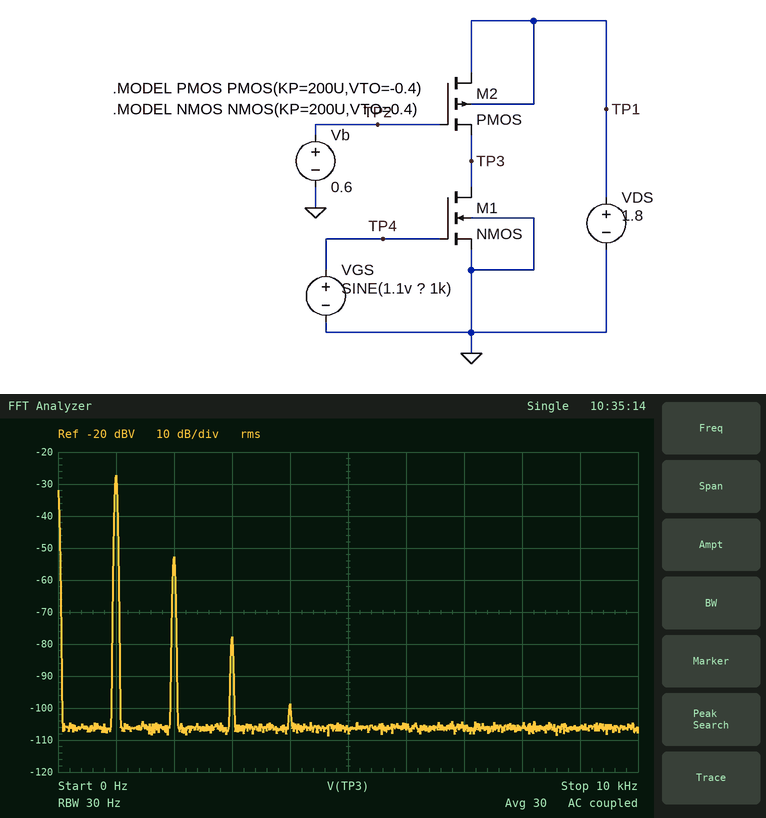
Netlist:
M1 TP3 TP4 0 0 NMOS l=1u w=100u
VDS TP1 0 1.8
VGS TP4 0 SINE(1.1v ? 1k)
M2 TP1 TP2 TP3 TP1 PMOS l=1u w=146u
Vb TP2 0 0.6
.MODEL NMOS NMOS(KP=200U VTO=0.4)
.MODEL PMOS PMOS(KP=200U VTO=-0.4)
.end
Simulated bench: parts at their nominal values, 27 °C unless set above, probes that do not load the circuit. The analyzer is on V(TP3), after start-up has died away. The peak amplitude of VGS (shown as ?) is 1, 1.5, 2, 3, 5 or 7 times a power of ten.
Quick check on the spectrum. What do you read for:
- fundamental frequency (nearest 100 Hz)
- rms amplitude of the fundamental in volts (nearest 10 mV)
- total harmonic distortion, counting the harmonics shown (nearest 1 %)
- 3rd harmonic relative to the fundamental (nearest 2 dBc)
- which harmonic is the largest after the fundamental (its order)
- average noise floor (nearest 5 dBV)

1.0 kHz
40 mV
5 %
-50 dBc
2
-105 dBV
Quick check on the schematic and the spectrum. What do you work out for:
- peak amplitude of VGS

70 mV
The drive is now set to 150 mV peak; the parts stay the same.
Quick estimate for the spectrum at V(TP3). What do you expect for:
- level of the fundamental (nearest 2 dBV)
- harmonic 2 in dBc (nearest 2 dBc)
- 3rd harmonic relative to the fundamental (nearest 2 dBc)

-20 dBV
-18 dBc
-36 dBc
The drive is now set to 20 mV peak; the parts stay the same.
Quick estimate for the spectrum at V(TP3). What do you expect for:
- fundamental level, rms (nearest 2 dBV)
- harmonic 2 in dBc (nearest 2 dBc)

-38 dBV
-36 dBc
